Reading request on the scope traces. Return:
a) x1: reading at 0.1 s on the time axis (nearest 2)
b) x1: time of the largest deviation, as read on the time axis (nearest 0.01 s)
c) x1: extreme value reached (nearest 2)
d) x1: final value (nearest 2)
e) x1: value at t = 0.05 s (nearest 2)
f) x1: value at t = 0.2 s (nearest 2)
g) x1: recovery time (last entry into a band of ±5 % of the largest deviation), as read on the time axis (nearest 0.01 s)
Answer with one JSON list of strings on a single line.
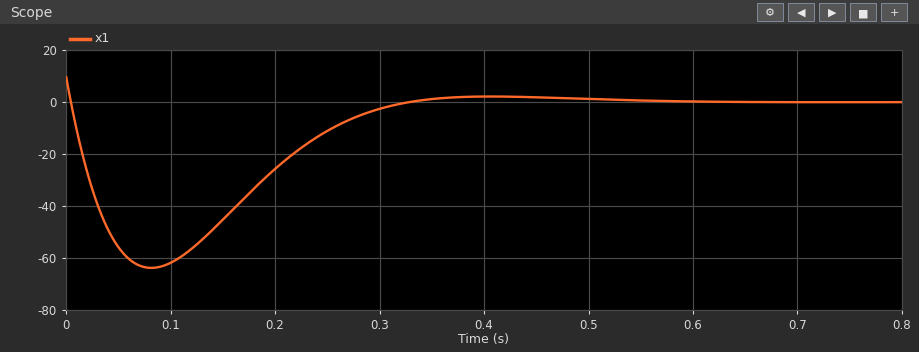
["-62", "0.08 s", "-64", "0", "-56", "-26", "0.29 s"]
